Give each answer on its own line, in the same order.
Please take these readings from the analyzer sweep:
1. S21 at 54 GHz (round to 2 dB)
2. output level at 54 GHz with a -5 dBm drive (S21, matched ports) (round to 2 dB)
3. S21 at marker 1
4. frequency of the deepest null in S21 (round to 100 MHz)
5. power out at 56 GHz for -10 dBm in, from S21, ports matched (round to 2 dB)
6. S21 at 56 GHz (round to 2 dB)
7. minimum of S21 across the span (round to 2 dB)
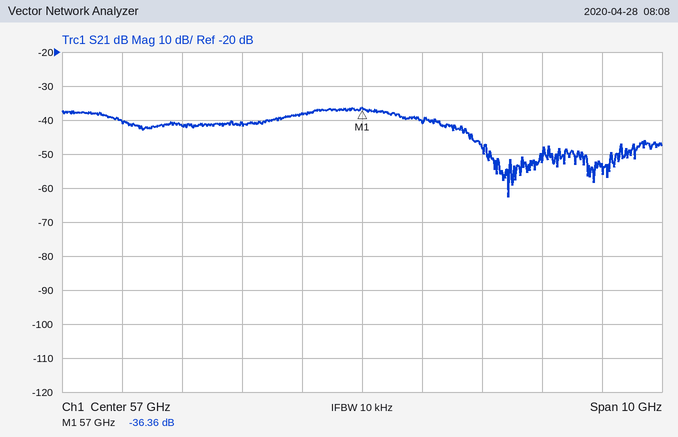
-42 dB
-46 dBm
-36.36 dB
59.4 GHz
-48 dBm
-38 dB
-62 dB
